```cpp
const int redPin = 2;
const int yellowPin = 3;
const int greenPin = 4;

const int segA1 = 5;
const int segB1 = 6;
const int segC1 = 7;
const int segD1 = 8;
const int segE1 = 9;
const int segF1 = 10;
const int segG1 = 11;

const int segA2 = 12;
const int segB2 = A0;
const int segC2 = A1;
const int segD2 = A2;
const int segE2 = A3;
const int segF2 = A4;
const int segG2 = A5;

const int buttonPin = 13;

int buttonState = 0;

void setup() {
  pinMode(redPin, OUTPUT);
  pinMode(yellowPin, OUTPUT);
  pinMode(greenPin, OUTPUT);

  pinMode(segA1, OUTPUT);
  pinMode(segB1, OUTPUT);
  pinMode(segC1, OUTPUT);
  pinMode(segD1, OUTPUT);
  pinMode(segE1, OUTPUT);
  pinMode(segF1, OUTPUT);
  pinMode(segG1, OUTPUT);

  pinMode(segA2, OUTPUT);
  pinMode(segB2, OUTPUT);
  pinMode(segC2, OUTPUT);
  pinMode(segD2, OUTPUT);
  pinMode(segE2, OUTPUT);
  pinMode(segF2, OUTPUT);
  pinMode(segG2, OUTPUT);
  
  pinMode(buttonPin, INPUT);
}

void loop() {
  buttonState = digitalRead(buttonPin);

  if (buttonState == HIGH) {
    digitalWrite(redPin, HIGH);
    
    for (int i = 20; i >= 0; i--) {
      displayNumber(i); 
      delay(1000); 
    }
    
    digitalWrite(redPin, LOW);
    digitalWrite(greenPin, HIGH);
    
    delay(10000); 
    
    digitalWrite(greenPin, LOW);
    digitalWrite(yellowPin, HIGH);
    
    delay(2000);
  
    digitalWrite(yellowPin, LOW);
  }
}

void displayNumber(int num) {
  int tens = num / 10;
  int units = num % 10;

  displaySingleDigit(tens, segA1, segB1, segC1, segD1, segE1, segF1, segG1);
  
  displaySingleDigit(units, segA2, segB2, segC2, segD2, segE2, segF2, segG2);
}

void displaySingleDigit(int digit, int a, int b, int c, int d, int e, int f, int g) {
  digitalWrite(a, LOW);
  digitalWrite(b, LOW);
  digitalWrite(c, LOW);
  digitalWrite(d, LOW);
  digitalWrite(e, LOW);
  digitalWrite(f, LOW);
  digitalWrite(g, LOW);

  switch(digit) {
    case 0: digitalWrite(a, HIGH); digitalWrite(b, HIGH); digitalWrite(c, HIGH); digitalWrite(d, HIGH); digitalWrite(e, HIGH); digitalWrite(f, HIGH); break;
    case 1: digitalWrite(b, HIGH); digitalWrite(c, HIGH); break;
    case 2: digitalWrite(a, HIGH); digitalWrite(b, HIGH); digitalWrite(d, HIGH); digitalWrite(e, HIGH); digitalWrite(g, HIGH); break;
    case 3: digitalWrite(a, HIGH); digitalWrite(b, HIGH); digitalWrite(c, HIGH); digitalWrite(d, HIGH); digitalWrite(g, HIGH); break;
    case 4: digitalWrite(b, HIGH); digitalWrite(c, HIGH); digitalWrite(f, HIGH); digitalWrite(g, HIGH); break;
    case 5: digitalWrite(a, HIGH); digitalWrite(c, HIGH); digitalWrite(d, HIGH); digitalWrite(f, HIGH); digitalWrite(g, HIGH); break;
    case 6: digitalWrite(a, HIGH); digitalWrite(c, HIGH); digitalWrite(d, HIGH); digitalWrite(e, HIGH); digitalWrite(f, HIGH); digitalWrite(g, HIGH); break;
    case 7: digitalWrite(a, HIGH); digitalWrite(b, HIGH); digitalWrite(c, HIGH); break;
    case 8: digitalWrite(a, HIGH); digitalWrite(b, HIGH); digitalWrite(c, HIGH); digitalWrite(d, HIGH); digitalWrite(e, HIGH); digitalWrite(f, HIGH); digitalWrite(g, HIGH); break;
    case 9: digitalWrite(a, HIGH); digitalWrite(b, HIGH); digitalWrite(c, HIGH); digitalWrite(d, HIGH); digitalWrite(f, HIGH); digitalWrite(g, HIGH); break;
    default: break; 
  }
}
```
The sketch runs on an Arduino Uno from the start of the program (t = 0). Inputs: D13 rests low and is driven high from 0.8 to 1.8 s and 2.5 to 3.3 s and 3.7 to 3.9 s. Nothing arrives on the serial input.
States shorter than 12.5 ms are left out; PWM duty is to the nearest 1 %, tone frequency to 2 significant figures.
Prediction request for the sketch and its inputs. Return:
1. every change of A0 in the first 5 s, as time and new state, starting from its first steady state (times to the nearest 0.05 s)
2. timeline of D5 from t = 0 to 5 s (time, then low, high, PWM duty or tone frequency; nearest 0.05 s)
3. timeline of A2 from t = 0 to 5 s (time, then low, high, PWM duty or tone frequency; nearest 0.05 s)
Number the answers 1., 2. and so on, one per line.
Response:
1. 0 s low; 0.8 s high; 4.8 s low
2. 0 s low; 0.8 s high; 1.8 s low
3. 0 s low; 0.8 s high; 3.8 s low; 4.8 s high
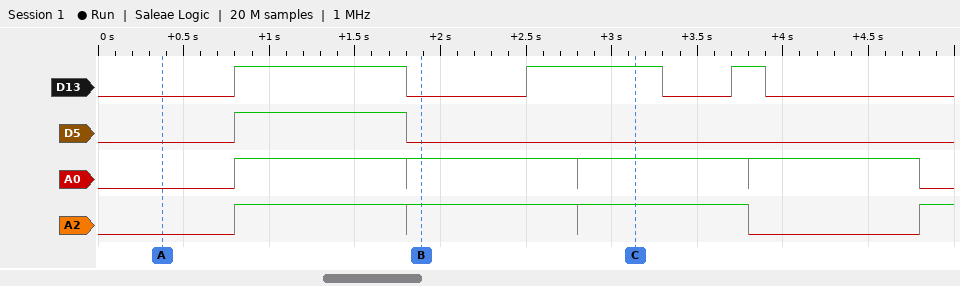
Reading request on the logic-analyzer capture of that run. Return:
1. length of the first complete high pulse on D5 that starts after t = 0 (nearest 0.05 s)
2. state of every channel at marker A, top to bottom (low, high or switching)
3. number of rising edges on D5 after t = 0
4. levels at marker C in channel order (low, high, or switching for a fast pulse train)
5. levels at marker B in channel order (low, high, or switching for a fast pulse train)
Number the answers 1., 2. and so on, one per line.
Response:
1. 1.00 s
2. D13 low, D5 low, A0 low, A2 low
3. 1
4. D13 high, D5 low, A0 high, A2 high
5. D13 low, D5 low, A0 high, A2 high
